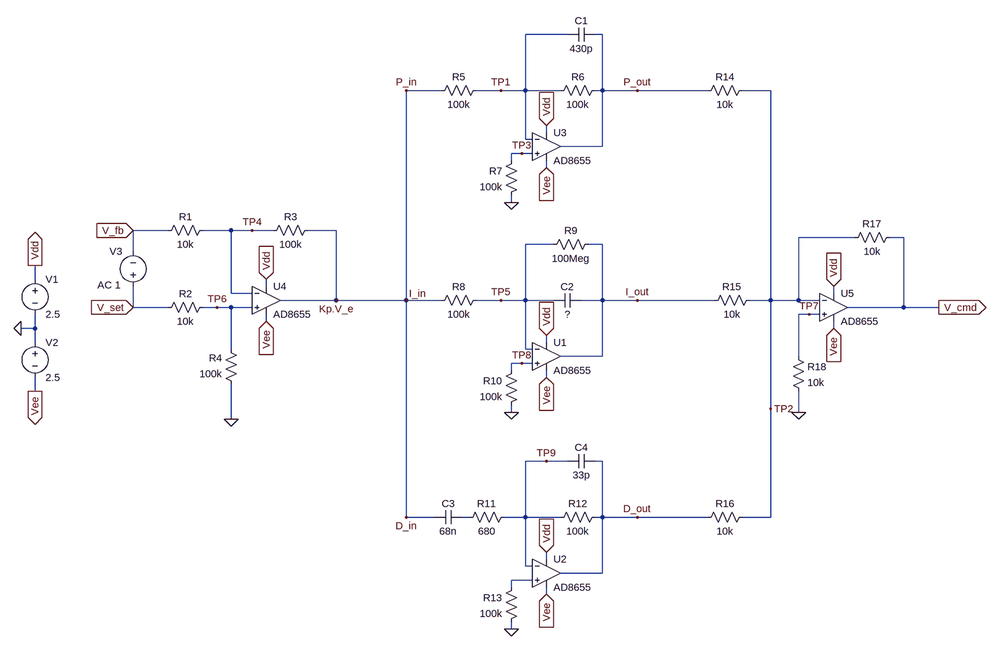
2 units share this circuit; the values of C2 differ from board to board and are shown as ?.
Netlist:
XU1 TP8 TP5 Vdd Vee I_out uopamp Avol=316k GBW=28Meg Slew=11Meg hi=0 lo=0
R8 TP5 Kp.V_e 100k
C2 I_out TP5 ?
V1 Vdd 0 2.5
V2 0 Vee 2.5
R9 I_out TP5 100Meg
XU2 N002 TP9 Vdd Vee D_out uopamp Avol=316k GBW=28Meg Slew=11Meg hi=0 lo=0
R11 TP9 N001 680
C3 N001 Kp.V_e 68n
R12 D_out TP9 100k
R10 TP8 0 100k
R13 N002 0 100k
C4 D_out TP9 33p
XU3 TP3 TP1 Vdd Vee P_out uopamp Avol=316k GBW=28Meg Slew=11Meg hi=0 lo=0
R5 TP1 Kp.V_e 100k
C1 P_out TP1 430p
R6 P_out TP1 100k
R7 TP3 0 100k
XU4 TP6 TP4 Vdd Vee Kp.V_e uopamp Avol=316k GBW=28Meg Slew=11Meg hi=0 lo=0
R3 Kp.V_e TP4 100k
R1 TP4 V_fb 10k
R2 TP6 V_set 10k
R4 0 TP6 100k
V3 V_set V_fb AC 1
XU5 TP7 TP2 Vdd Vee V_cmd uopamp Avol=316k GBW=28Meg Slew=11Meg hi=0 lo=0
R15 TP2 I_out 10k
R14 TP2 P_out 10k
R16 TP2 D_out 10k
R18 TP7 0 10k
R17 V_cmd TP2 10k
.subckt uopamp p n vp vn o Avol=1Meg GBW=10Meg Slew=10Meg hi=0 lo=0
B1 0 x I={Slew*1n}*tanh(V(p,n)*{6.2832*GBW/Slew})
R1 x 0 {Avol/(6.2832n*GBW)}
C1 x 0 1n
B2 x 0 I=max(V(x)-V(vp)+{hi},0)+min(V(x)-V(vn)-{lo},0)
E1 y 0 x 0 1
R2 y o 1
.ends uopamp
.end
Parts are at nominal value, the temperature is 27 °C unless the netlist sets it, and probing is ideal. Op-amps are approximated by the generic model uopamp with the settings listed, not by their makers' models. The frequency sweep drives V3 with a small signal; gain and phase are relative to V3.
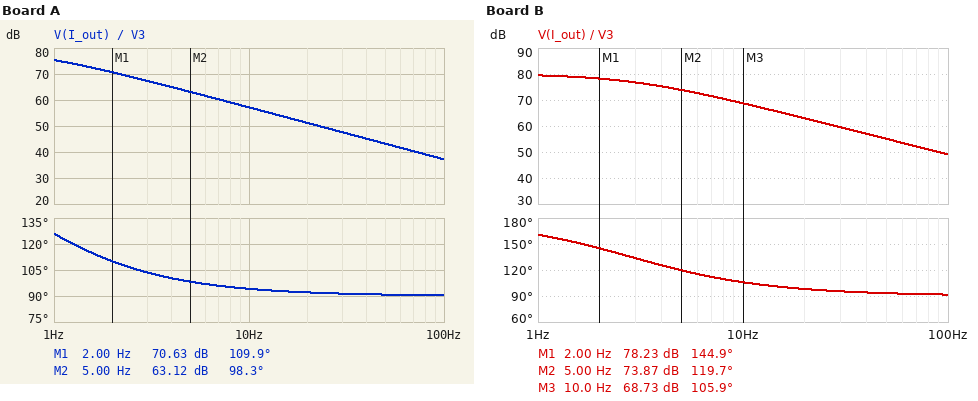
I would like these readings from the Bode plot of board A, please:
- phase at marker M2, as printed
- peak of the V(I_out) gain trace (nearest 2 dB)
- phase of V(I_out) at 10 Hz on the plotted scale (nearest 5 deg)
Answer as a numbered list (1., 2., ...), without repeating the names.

1. 98.3 deg
2. 76 dB
3. 95 deg
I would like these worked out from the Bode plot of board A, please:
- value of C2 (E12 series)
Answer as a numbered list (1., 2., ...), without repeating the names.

1. 2.2 nF
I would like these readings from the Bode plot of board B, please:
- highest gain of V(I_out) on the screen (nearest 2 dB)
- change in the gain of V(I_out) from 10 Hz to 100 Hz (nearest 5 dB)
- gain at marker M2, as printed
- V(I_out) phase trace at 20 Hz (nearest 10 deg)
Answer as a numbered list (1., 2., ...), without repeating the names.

1. 80 dB
2. -20 dB
3. 73.87 dB
4. 100 deg
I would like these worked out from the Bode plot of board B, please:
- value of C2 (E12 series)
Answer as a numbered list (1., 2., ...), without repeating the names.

1. 560 pF
